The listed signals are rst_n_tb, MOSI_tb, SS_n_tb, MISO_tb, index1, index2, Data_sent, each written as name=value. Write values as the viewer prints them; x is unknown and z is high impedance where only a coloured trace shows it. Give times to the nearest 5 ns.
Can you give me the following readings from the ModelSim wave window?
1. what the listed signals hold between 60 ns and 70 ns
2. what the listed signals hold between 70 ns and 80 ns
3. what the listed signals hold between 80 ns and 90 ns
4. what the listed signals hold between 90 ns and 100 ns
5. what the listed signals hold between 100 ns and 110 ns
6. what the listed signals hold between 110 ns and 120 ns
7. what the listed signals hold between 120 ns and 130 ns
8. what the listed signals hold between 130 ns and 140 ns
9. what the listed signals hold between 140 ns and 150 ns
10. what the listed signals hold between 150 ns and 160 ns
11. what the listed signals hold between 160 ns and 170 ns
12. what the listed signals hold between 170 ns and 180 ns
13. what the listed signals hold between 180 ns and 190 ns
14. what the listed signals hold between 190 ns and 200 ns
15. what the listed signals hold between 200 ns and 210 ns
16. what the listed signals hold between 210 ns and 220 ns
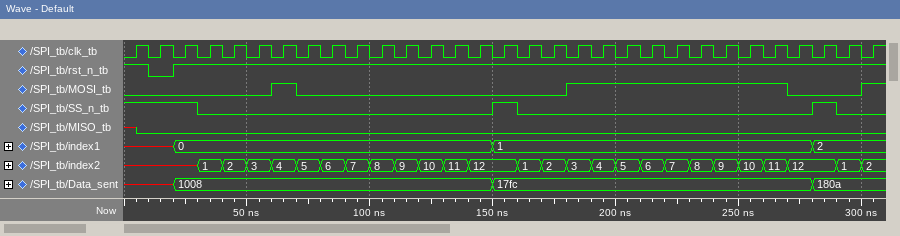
rst_n_tb=1, MOSI_tb=1, SS_n_tb=0, MISO_tb=0, index1=0, index2=4, Data_sent=1008
rst_n_tb=1, MOSI_tb=0, SS_n_tb=0, MISO_tb=0, index1=0, index2=5, Data_sent=1008
rst_n_tb=1, MOSI_tb=0, SS_n_tb=0, MISO_tb=0, index1=0, index2=6, Data_sent=1008
rst_n_tb=1, MOSI_tb=0, SS_n_tb=0, MISO_tb=0, index1=0, index2=7, Data_sent=1008
rst_n_tb=1, MOSI_tb=0, SS_n_tb=0, MISO_tb=0, index1=0, index2=8, Data_sent=1008
rst_n_tb=1, MOSI_tb=0, SS_n_tb=0, MISO_tb=0, index1=0, index2=9, Data_sent=1008
rst_n_tb=1, MOSI_tb=0, SS_n_tb=0, MISO_tb=0, index1=0, index2=10, Data_sent=1008
rst_n_tb=1, MOSI_tb=0, SS_n_tb=0, MISO_tb=0, index1=0, index2=11, Data_sent=1008
rst_n_tb=1, MOSI_tb=0, SS_n_tb=0, MISO_tb=0, index1=0, index2=12, Data_sent=1008
rst_n_tb=1, MOSI_tb=0, SS_n_tb=1, MISO_tb=0, index1=1, index2=12, Data_sent=17fc
rst_n_tb=1, MOSI_tb=0, SS_n_tb=0, MISO_tb=0, index1=1, index2=1, Data_sent=17fc
rst_n_tb=1, MOSI_tb=0, SS_n_tb=0, MISO_tb=0, index1=1, index2=2, Data_sent=17fc
rst_n_tb=1, MOSI_tb=1, SS_n_tb=0, MISO_tb=0, index1=1, index2=3, Data_sent=17fc
rst_n_tb=1, MOSI_tb=1, SS_n_tb=0, MISO_tb=0, index1=1, index2=4, Data_sent=17fc
rst_n_tb=1, MOSI_tb=1, SS_n_tb=0, MISO_tb=0, index1=1, index2=5, Data_sent=17fc
rst_n_tb=1, MOSI_tb=1, SS_n_tb=0, MISO_tb=0, index1=1, index2=6, Data_sent=17fc
